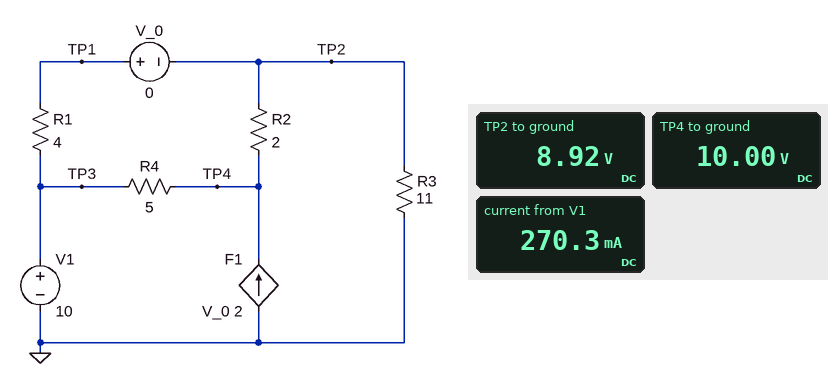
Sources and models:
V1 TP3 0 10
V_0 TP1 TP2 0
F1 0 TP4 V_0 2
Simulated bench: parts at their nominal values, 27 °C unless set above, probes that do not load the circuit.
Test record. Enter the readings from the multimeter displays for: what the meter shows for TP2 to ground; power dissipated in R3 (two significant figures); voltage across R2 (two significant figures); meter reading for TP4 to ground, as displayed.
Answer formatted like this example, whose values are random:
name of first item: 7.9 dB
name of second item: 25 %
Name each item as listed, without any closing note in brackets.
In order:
what the meter shows for TP2 to ground: 8.92 V
power dissipated in R3: 7.2 W
voltage across R2: 1.1 V
meter reading for TP4 to ground, as displayed: 10.00 V
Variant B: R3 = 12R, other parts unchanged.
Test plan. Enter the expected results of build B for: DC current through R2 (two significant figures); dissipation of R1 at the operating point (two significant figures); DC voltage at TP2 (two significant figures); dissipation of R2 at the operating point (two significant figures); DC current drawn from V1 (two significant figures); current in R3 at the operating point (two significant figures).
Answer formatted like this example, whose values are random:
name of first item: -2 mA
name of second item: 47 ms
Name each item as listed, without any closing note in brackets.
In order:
DC current through R2: 500 mA
dissipation of R1 at the operating point: 250 mW
DC voltage at TP2: 9.0 V
dissipation of R2 at the operating point: 500 mW
DC current drawn from V1: 250 mA
current in R3 at the operating point: 750 mA
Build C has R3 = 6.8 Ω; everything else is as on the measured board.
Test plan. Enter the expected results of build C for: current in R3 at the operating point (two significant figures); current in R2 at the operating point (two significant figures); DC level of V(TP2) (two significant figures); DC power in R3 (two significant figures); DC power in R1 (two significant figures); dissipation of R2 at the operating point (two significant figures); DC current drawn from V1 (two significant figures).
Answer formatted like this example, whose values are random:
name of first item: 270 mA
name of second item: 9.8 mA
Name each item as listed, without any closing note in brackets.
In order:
current in R3 at the operating point: 1.2 A
current in R2 at the operating point: 820 mA
DC level of V(TP2): 8.4 V
DC power in R3: 10 W
DC power in R1: 670 mW
dissipation of R2 at the operating point: 1.3 W
DC current drawn from V1: 410 mA
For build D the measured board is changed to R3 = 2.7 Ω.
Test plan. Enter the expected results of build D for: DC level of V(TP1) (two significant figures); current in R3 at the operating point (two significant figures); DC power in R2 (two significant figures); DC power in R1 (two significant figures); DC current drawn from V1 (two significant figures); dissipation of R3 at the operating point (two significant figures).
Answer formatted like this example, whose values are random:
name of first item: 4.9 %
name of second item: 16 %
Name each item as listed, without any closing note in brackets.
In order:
DC level of V(TP1): 6.7 V
current in R3 at the operating point: 2.5 A
DC power in R2: 5.5 W
DC power in R1: 2.7 W
DC current drawn from V1: 830 mA
dissipation of R3 at the operating point: 17 W
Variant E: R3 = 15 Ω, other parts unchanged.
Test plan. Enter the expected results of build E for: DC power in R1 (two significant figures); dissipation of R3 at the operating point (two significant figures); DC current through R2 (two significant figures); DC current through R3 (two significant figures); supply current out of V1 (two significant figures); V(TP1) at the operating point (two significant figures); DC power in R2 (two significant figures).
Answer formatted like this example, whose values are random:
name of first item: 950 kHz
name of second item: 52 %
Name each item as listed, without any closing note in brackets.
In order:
DC power in R1: 170 mW
dissipation of R3 at the operating point: 5.6 W
DC current through R2: 410 mA
DC current through R3: 610 mA
supply current out of V1: 200 mA
V(TP1) at the operating point: 9.2 V
DC power in R2: 330 mW
